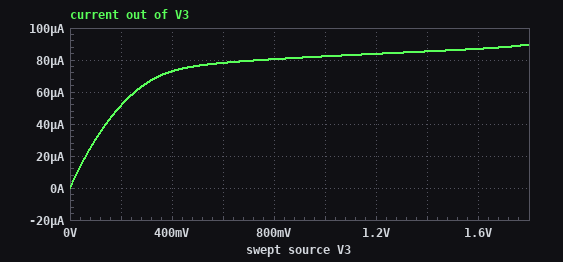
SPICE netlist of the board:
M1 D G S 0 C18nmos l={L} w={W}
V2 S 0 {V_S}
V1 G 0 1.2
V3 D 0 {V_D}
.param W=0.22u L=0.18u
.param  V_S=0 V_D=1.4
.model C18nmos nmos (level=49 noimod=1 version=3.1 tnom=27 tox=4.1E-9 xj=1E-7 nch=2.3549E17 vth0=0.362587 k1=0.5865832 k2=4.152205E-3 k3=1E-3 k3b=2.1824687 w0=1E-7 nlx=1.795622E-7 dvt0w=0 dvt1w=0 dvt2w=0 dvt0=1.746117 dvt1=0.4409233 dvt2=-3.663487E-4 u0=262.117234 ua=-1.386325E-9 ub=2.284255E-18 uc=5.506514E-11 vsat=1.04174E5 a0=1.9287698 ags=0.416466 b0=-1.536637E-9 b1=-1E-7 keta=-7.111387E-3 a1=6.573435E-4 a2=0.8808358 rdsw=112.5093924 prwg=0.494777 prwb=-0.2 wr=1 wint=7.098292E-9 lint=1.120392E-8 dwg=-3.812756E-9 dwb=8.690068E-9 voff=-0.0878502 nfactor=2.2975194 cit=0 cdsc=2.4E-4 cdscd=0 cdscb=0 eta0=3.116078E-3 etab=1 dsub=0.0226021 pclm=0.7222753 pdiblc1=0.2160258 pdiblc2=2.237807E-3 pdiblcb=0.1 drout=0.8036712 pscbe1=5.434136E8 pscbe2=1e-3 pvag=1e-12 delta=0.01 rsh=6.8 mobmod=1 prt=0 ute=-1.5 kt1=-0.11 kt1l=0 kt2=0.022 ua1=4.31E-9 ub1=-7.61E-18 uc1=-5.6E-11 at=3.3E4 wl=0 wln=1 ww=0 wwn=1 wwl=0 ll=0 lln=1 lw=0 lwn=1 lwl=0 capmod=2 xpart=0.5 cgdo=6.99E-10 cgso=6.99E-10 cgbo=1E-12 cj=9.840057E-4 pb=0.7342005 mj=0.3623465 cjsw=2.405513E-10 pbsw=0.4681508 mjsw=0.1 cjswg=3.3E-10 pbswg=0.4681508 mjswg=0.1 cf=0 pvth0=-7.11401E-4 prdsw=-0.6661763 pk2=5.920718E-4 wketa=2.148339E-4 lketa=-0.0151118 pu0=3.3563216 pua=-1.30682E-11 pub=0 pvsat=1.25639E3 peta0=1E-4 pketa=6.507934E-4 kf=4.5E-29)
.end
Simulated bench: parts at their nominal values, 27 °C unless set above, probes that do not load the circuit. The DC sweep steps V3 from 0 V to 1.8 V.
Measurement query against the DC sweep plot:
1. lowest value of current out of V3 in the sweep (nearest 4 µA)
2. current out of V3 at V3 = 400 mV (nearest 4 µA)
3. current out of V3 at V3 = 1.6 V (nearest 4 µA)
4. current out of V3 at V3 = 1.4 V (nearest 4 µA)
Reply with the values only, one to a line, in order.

0 A
72 µA
88 µA
84 µA
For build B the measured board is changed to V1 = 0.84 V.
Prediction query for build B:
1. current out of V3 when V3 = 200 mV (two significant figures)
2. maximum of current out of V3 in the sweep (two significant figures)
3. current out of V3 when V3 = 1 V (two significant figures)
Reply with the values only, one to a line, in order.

24 µA
38 µA
32 µA
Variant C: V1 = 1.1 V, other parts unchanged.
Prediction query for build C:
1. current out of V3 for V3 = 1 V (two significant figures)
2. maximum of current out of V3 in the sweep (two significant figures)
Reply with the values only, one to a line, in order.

68 µA
75 µA
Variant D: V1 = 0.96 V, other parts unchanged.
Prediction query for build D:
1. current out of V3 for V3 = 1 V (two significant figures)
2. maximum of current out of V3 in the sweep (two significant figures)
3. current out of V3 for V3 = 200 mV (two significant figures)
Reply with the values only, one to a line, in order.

48 µA
55 µA
34 µA
